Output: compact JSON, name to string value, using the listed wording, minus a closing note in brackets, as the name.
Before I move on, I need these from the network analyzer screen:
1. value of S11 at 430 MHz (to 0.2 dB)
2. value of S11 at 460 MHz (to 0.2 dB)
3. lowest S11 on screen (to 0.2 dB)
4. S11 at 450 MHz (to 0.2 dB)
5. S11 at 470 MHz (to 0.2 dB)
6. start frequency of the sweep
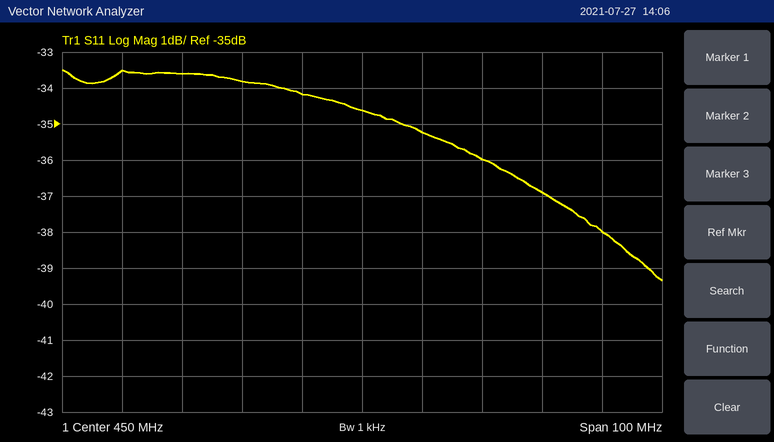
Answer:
{"value of S11 at 430 MHz": "-33.8 dB", "value of S11 at 460 MHz": "-35.2 dB", "lowest S11 on screen": "-39.4 dB", "S11 at 450 MHz": "-34.6 dB", "S11 at 470 MHz": "-36.0 dB", "start frequency of the sweep": "400 MHz"}
